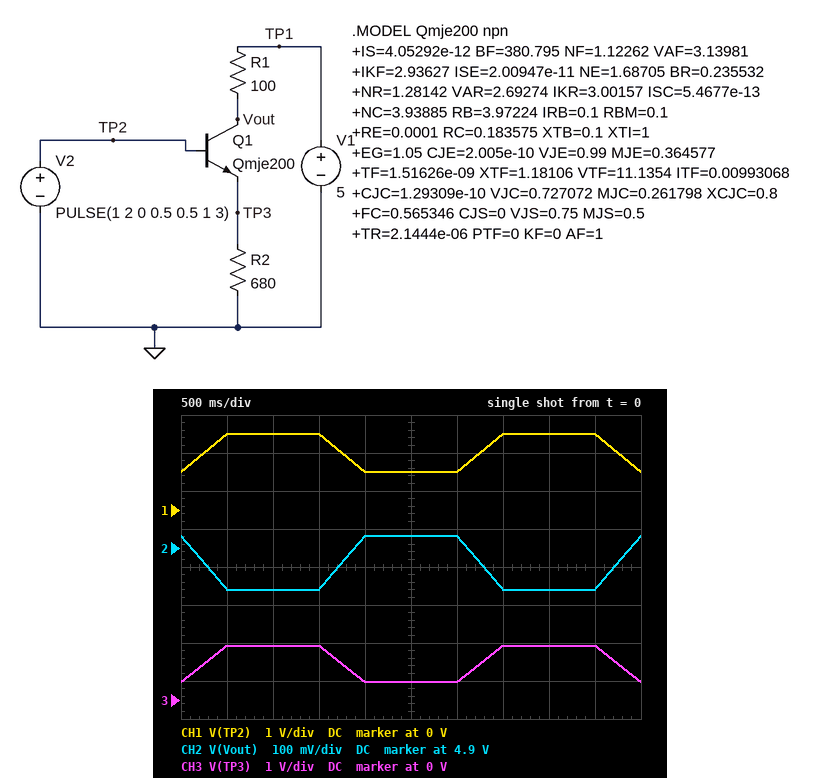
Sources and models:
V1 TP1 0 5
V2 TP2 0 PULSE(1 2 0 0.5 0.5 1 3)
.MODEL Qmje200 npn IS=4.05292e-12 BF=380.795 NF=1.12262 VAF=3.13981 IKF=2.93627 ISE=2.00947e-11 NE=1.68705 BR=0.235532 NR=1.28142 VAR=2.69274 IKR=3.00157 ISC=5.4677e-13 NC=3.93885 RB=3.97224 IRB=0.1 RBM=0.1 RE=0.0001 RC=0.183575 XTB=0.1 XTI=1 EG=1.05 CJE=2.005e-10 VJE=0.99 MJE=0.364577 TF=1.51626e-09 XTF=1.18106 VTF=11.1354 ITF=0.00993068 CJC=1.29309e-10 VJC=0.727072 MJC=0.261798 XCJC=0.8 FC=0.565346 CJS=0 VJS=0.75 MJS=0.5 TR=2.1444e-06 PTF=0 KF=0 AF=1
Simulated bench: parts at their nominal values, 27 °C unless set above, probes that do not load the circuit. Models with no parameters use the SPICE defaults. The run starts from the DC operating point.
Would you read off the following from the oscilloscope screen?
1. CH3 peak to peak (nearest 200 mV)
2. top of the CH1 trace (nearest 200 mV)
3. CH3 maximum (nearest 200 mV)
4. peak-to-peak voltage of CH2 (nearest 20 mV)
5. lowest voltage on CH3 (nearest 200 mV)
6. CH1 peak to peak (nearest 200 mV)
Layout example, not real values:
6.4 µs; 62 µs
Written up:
1.0 V; 2.0 V; 1.4 V; 140 mV; 400 mV; 1.0 V
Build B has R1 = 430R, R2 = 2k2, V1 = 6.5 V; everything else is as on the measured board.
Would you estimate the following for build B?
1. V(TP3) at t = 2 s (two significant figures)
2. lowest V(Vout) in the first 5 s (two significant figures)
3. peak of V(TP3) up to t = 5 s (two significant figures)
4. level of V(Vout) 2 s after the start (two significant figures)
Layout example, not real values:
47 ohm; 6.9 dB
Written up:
510 mV; 6.2 V; 1.5 V; 6.4 V
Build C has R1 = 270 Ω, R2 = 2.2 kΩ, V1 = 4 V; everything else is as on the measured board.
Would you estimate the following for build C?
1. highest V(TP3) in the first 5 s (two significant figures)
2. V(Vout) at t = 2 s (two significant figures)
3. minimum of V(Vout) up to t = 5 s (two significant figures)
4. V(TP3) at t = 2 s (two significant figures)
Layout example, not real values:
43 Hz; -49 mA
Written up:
1.5 V; 3.9 V; 3.8 V; 500 mV
